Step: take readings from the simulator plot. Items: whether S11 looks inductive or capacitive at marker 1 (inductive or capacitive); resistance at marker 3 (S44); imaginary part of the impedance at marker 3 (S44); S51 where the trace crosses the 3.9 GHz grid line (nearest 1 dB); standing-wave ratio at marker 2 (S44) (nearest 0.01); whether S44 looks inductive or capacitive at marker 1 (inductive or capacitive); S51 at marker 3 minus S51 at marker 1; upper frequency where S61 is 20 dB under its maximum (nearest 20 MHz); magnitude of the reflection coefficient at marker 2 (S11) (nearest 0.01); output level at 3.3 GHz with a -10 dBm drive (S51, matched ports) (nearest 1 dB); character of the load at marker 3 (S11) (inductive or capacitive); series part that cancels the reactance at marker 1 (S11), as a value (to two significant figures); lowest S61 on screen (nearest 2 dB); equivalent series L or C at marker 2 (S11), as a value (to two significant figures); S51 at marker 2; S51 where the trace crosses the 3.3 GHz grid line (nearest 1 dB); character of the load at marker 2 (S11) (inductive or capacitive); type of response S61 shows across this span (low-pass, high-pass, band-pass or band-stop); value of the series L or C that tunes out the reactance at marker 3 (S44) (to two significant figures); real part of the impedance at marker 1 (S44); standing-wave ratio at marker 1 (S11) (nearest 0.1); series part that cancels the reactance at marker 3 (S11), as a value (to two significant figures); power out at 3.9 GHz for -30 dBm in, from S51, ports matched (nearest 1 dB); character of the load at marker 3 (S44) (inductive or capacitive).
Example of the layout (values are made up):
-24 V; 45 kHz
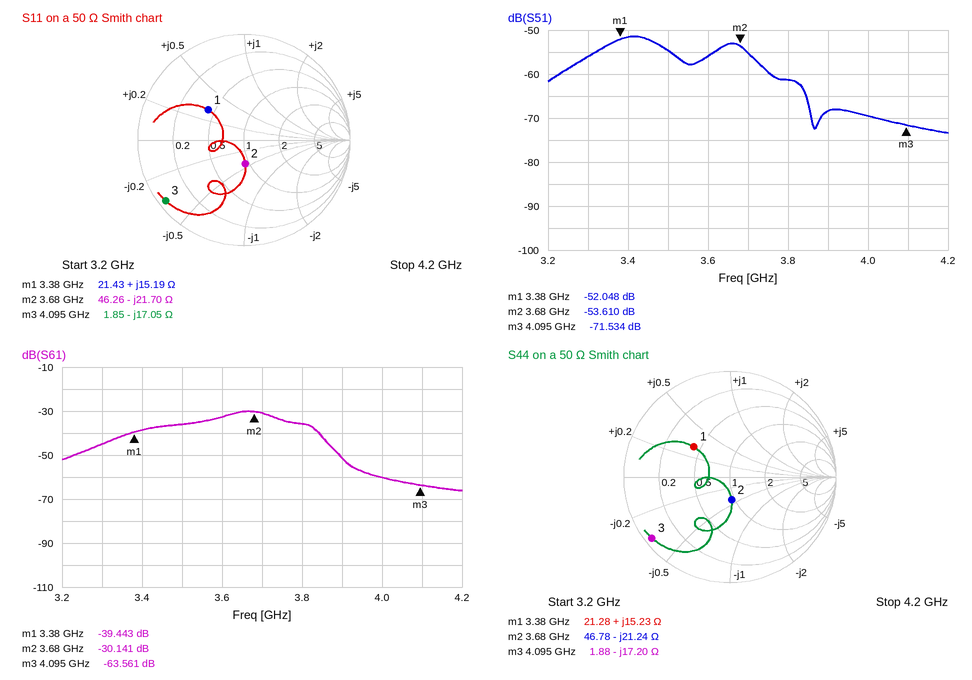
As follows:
inductive; 1.88 Ω; -17.20 Ω; -68 dB; 1.55; inductive; -19.486 dB; 3.90 GHz; 0.22; -66 dBm; capacitive; 3.1 pF; -66 dB; 2.0 pF; -53.610 dB; -56 dB; capacitive; band-pass; 670 pH; 21.28 Ω; 2.6; 660 pH; -98 dBm; capacitive
